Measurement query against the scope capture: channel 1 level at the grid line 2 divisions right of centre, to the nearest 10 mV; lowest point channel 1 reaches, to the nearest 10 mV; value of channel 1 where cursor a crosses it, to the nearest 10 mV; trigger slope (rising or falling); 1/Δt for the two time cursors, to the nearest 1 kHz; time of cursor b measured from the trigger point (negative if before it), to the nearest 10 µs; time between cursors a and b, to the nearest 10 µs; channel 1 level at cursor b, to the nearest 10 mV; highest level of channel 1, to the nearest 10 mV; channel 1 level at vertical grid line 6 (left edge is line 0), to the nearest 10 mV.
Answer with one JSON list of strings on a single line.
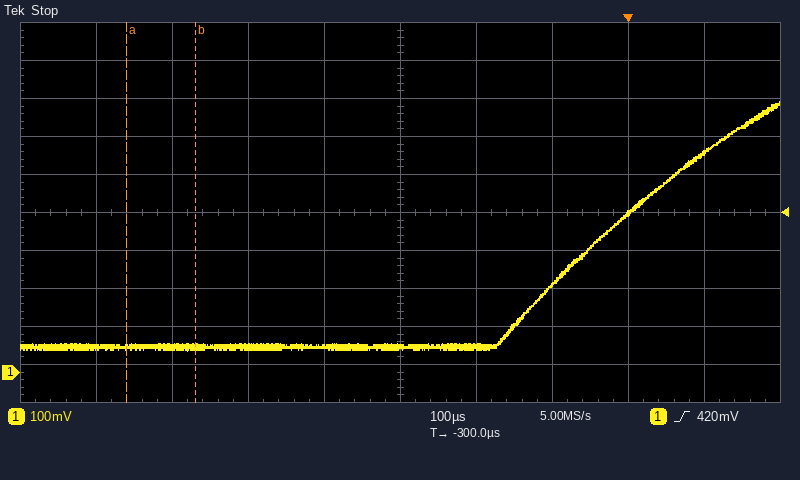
["230 mV", "60 mV", "70 mV", "rising", "11 kHz", "-570 µs", "90 µs", "70 mV", "710 mV", "70 mV"]
